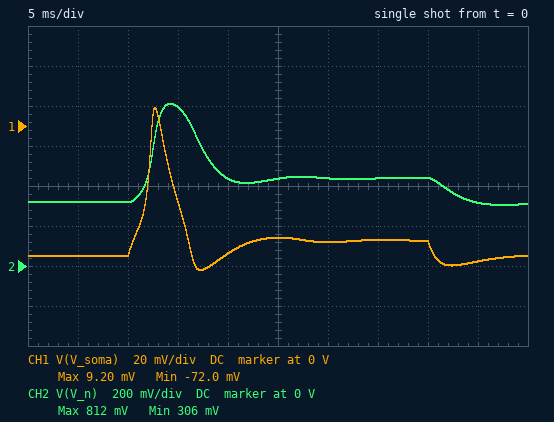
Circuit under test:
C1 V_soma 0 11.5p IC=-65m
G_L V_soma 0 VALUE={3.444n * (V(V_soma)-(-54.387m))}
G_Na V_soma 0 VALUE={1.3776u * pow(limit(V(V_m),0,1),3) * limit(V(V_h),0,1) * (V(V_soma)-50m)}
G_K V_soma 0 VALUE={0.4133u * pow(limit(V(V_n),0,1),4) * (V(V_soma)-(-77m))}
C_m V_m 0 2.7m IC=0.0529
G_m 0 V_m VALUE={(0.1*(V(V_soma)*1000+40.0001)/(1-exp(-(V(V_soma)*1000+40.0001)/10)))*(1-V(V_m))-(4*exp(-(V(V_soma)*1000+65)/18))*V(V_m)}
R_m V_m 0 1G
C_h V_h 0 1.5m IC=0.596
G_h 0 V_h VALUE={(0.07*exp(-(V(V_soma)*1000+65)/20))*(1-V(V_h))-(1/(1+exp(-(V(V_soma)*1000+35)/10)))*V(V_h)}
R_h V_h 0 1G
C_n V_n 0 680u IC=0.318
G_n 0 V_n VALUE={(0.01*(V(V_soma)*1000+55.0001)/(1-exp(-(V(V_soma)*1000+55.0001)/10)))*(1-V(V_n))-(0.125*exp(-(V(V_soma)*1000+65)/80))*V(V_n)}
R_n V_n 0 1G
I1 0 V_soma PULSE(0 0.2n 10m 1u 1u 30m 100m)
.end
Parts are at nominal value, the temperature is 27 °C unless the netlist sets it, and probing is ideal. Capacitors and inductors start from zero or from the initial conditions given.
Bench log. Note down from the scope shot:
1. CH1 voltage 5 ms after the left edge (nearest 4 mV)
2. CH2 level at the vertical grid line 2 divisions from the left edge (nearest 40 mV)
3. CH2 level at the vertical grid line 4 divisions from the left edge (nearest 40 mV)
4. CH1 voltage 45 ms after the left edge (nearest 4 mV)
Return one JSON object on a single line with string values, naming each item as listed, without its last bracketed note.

{"CH1 voltage 5 ms after the left edge": "-64 mV", "CH2 level at the vertical grid line 2 divisions from the left edge": "320 mV", "CH2 level at the vertical grid line 4 divisions from the left edge": "440 mV", "CH1 voltage 45 ms after the left edge": "-68 mV"}
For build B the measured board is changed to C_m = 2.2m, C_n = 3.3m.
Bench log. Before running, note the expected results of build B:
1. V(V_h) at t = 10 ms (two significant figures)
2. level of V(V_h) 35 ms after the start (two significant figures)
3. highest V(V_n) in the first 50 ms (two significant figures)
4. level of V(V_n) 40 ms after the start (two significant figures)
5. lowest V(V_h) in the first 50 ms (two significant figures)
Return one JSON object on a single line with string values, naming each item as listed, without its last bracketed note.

{"V(V_h) at t = 10 ms": "600 mV", "level of V(V_h) 35 ms after the start": "490 mV", "highest V(V_n) in the first 50 ms": "680 mV", "level of V(V_n) 40 ms after the start": "450 mV", "lowest V(V_h) in the first 50 ms": "45 mV"}
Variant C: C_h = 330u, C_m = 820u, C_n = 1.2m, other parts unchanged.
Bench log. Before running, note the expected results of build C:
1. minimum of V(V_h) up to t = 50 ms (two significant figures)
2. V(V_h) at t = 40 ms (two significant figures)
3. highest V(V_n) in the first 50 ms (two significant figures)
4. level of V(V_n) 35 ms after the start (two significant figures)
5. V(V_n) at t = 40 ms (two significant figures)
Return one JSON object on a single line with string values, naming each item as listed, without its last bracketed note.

{"minimum of V(V_h) up to t = 50 ms": "21 mV", "V(V_h) at t = 40 ms": "510 mV", "highest V(V_n) in the first 50 ms": "620 mV", "level of V(V_n) 35 ms after the start": "560 mV", "V(V_n) at t = 40 ms": "430 mV"}
